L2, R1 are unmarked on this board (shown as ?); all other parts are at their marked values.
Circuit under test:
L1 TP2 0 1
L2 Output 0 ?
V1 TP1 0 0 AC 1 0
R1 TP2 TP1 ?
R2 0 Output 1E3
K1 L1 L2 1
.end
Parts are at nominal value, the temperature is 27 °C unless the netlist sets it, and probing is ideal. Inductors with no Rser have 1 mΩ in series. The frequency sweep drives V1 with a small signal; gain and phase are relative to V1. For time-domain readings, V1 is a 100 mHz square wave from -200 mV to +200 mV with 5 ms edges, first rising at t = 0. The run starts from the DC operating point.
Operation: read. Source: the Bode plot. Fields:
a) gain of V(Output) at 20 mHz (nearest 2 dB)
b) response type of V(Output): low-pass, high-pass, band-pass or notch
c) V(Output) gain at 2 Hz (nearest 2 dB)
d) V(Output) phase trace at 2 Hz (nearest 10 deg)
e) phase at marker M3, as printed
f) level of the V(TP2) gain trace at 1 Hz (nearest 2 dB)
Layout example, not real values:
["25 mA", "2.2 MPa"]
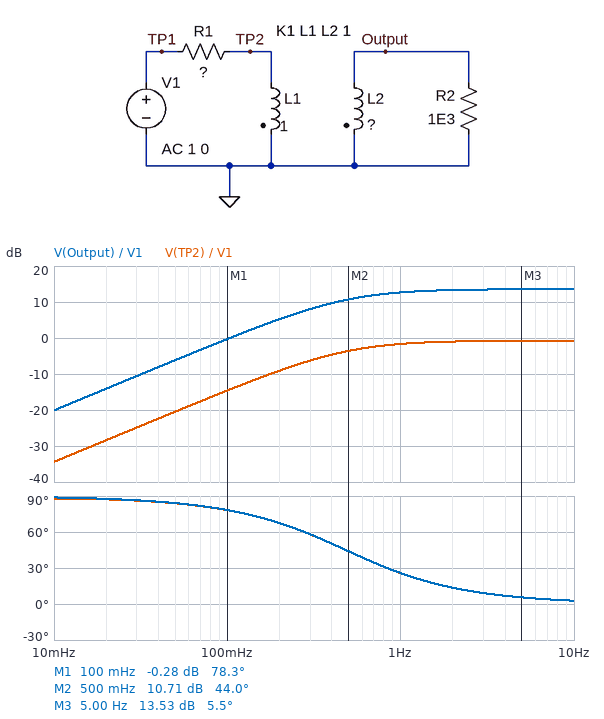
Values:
["-14 dB", "high-pass", "14 dB", "10 deg", "5.5 deg", "-2 dB"]
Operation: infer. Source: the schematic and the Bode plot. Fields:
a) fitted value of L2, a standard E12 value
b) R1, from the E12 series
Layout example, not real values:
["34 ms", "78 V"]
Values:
["27 H", "3.3 Ω"]
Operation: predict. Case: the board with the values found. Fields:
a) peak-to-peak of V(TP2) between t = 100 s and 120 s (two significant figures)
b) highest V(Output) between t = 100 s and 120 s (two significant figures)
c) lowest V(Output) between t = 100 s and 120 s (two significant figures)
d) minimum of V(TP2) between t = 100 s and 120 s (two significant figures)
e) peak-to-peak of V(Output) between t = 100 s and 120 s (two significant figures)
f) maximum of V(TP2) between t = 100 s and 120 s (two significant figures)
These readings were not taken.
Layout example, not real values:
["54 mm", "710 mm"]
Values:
["730 mV", "1.9 V", "-1.9 V", "-360 mV", "3.8 V", "360 mV"]
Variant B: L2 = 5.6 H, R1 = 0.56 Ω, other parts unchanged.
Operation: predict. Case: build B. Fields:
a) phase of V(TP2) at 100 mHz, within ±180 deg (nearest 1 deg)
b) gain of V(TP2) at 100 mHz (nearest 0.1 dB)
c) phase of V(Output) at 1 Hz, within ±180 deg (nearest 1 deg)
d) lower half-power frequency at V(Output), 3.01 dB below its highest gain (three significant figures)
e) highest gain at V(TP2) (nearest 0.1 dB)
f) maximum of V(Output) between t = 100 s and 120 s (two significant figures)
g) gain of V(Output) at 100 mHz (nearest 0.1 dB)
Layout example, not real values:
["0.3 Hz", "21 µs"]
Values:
["42 deg", "-2.6 dB", "5 deg", "89.0 mHz", "0 dB", "890 mV", "4.9 dB"]
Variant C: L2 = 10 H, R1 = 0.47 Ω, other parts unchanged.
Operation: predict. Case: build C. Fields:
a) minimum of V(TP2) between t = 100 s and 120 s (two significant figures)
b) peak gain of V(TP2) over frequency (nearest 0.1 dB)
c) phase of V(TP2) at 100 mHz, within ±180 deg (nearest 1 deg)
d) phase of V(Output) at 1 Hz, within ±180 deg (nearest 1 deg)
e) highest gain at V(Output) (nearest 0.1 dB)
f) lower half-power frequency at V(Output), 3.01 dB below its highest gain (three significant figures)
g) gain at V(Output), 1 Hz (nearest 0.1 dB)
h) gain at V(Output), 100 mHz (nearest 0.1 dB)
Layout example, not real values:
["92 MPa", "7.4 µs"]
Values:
["-360 mV", "0 dB", "37 deg", "4 deg", "10.0 dB", "74.6 mHz", "9.9 dB", "8.0 dB"]
